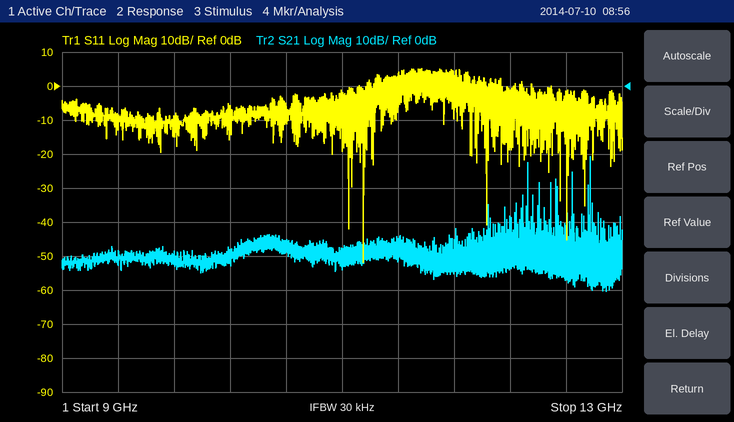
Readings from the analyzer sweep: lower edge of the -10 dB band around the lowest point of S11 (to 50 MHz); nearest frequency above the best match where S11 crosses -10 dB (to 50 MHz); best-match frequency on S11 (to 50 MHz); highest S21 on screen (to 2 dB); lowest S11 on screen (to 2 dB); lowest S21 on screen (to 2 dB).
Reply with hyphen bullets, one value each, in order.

- 11.15 GHz
- 11.15 GHz
- 11.15 GHz
- -20 dB
- -52 dB
- -60 dB
